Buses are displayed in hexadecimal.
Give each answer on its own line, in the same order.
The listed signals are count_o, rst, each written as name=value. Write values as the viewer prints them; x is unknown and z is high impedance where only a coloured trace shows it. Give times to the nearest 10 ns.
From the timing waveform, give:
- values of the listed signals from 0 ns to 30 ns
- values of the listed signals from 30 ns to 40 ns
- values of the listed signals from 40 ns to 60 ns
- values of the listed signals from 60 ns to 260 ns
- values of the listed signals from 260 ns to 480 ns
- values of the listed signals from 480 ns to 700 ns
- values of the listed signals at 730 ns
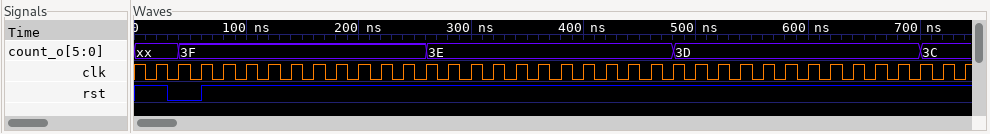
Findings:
count_o=xx, rst=1
count_o=xx, rst=0
count_o=3F, rst=0
count_o=3F, rst=1
count_o=3E, rst=1
count_o=3D, rst=1
count_o=3C, rst=1
